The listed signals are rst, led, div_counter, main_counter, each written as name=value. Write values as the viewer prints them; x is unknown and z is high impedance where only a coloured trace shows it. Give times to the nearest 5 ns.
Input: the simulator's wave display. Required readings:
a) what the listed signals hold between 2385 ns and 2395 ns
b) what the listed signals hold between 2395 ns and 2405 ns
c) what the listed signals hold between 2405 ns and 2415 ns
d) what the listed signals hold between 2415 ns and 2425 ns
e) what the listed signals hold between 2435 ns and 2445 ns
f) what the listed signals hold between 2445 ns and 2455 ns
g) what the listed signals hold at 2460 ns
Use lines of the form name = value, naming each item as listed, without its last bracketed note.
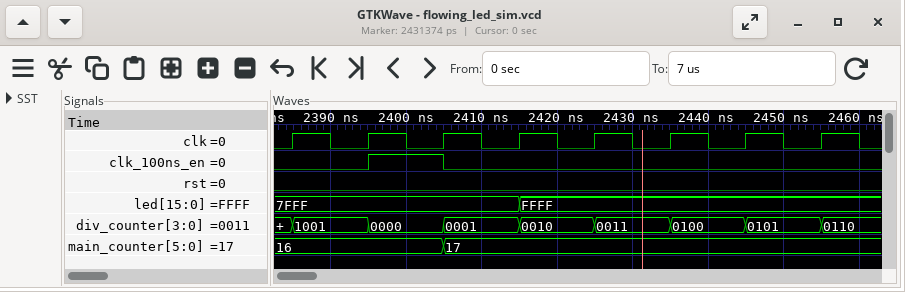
what the listed signals hold between 2385 ns and 2395 ns = rst=0, led=7FFF, div_counter=1001, main_counter=16
what the listed signals hold between 2395 ns and 2405 ns = rst=0, led=7FFF, div_counter=0000, main_counter=16
what the listed signals hold between 2405 ns and 2415 ns = rst=0, led=7FFF, div_counter=0001, main_counter=17
what the listed signals hold between 2415 ns and 2425 ns = rst=0, led=FFFF, div_counter=0010, main_counter=17
what the listed signals hold between 2435 ns and 2445 ns = rst=0, led=FFFF, div_counter=0100, main_counter=17
what the listed signals hold between 2445 ns and 2455 ns = rst=0, led=FFFF, div_counter=0101, main_counter=17
what the listed signals hold at 2460 ns = rst=0, led=FFFF, div_counter=0110, main_counter=17
